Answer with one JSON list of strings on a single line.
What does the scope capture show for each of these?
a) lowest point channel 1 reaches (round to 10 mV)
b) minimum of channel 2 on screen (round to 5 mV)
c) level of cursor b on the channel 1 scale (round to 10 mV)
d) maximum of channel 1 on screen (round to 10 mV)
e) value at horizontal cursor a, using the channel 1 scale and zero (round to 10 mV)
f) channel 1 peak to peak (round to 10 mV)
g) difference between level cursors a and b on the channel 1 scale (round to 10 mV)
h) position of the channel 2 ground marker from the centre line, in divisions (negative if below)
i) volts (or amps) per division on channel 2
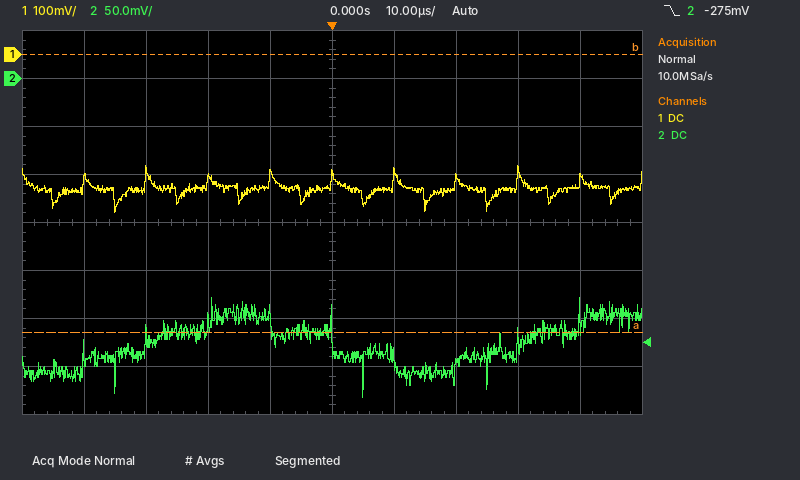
["-330 mV", "-330 mV", "0 mV", "-230 mV", "-580 mV", "100 mV", "580 mV", "+3.0 div", "50 mV"]
